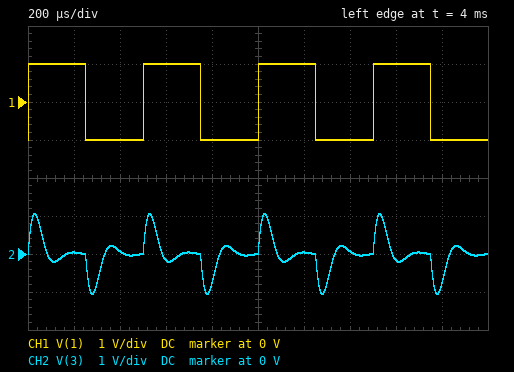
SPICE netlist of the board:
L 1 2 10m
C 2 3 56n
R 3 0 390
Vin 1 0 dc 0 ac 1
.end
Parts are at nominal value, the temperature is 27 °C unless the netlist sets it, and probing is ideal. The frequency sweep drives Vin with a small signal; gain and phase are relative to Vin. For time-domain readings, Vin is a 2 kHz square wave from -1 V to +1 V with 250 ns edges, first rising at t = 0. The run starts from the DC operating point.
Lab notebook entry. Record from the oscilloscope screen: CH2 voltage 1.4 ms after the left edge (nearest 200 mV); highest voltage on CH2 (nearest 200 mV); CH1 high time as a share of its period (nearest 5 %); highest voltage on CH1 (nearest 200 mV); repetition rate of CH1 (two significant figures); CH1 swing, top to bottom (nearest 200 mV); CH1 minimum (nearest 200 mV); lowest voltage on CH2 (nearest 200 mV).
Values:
0 V
1.0 V
50 %
1.0 V
2.0 kHz
2.0 V
-1.0 V
-1.0 V
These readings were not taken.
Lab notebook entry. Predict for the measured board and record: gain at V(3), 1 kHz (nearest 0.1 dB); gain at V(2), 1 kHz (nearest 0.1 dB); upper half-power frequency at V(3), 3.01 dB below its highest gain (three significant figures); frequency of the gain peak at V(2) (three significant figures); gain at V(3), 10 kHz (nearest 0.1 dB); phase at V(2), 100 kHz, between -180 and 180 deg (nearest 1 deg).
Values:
-17.1 dB
0.2 dB
10.5 kHz
5.85 kHz
-2.5 dB
-91 deg
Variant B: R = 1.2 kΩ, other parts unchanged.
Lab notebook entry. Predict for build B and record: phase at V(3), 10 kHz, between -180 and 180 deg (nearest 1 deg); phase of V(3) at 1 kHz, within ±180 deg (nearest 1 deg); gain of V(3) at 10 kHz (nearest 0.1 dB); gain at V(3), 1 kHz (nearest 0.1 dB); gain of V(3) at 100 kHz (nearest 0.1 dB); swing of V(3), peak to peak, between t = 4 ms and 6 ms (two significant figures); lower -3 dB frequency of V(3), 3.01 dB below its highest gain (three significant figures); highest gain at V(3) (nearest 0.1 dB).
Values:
-16 deg
67 deg
-0.3 dB
-8.0 dB
-14.5 dB
3.2 V
2.13 kHz
0 dB
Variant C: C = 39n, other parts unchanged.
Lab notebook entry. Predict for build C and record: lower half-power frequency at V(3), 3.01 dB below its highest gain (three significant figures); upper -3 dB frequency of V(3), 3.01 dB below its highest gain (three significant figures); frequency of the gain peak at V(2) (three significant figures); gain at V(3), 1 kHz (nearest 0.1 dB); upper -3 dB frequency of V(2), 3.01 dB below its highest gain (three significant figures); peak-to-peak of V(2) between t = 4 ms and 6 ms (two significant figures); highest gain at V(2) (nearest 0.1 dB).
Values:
5.53 kHz
11.7 kHz
7.24 kHz
-20.3 dB
10.3 kHz
3.5 V
4.6 dB
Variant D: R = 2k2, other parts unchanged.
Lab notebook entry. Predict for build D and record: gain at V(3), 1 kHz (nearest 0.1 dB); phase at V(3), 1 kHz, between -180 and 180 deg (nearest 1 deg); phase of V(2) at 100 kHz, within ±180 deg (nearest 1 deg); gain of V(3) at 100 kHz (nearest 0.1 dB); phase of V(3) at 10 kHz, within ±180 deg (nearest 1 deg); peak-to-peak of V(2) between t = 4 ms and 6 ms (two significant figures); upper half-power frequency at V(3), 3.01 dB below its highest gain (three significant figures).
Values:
-4.1 dB
52 deg
-71 deg
-9.6 dB
-9 deg
2.1 V
36.3 kHz
